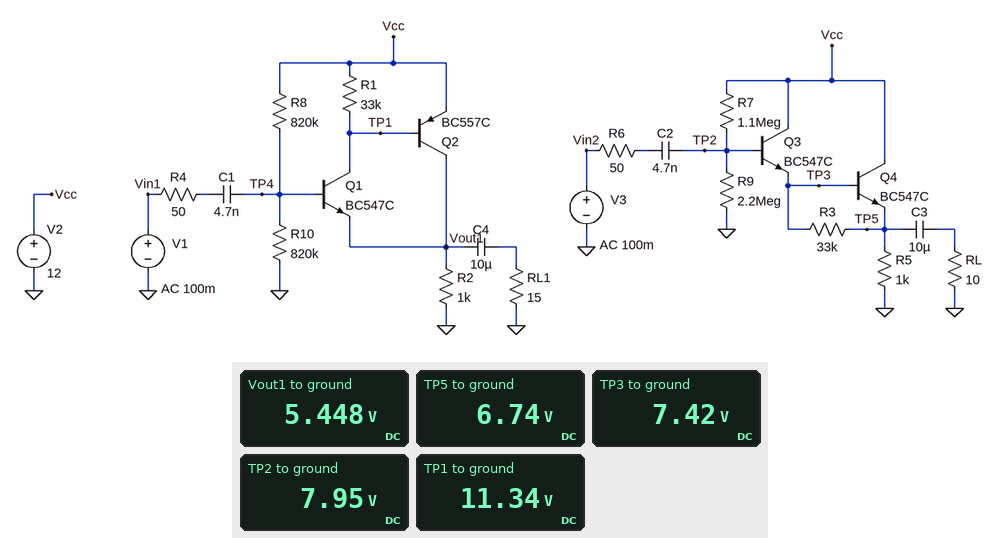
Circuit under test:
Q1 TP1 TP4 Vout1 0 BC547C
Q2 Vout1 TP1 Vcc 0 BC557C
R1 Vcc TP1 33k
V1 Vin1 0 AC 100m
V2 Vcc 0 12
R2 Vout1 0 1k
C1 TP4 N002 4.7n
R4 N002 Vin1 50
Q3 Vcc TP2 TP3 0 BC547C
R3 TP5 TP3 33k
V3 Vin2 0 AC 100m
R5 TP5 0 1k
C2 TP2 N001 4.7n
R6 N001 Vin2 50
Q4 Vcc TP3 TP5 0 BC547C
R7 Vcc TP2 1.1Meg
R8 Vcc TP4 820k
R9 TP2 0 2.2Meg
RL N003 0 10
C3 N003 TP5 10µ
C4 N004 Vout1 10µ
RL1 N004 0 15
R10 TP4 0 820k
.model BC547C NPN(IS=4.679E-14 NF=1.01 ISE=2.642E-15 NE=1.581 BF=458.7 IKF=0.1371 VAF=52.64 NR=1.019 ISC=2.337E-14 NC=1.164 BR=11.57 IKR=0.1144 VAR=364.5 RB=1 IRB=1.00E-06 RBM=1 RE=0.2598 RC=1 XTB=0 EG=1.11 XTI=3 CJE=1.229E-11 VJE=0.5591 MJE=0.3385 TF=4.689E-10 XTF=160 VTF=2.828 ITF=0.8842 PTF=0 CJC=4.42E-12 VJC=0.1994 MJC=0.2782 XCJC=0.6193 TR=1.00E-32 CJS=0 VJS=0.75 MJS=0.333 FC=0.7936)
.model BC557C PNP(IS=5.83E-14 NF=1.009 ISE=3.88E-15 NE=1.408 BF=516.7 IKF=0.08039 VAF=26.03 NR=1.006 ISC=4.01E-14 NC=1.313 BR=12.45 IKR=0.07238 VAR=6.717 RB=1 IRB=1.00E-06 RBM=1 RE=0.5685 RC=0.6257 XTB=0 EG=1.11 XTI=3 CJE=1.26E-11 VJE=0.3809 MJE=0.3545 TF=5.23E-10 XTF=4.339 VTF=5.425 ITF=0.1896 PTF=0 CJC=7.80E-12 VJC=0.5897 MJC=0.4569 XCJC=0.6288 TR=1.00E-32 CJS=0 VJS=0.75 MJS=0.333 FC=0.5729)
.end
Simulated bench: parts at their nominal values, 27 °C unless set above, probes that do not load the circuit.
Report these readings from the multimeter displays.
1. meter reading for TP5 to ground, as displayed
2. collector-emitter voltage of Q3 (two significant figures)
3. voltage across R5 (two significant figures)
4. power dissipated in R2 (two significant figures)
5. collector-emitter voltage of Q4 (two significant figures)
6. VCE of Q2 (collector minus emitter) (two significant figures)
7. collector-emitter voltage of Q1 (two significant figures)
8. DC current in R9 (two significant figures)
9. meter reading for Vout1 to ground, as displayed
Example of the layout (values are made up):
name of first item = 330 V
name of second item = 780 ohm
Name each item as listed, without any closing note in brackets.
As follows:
meter reading for TP5 to ground, as displayed = 6.74 V
collector-emitter voltage of Q3 = 4.6 V
voltage across R5 = 6.7 V
power dissipated in R2 = 30 mW
collector-emitter voltage of Q4 = 5.3 V
VCE of Q2 (collector minus emitter) = -6.6 V
collector-emitter voltage of Q1 = 5.9 V
DC current in R9 = 3.6 µA
meter reading for Vout1 to ground, as displayed = 5.448 V
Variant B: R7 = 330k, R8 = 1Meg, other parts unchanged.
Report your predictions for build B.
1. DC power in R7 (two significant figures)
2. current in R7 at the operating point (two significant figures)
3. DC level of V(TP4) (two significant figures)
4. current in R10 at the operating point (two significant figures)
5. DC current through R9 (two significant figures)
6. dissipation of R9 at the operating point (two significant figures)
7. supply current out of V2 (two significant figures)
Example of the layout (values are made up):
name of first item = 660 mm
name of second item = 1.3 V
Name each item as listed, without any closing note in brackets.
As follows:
DC power in R7 = 7.7 µW
current in R7 at the operating point = 4.8 µA
DC level of V(TP4) = 5.4 V
current in R10 at the operating point = 6.6 µA
DC current through R9 = 4.7 µA
dissipation of R9 at the operating point = 49 µW
supply current out of V2 = 14 mA
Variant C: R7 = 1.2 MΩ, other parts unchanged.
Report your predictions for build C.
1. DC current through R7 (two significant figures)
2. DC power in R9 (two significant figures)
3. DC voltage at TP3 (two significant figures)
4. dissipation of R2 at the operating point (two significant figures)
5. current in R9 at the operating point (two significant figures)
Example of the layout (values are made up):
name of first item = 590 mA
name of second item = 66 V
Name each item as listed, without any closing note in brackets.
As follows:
DC current through R7 = 3.6 µA
DC power in R9 = 27 µW
DC voltage at TP3 = 7.2 V
dissipation of R2 at the operating point = 30 mW
current in R9 at the operating point = 3.5 µA
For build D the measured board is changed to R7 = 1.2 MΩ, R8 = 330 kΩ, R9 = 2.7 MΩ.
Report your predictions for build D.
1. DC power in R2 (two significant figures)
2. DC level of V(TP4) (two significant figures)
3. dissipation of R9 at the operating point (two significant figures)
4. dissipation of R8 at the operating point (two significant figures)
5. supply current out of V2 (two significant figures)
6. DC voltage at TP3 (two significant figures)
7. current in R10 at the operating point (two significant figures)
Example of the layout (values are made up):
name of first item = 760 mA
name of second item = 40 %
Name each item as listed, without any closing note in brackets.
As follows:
DC power in R2 = 64 mW
DC level of V(TP4) = 8.5 V
dissipation of R9 at the operating point = 25 µW
dissipation of R8 at the operating point = 36 µW
supply current out of V2 = 15 mA
DC voltage at TP3 = 7.7 V
current in R10 at the operating point = 10 µA
